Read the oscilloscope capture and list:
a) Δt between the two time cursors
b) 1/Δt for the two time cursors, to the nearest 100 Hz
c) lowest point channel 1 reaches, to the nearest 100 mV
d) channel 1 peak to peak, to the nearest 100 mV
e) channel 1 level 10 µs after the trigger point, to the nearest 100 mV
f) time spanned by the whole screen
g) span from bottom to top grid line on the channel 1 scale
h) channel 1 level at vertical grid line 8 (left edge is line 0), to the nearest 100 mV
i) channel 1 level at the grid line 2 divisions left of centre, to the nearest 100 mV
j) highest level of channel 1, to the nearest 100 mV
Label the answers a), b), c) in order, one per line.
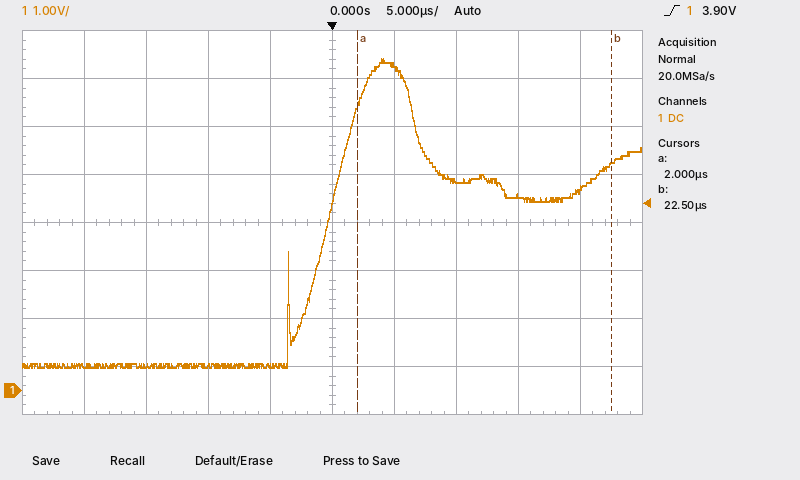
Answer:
a) 20.5 µs
b) 48.8 kHz
c) 500 mV
d) 6.4 V
e) 4.4 V
f) 50 µs
g) 8 V
h) 4.1 V
i) 500 mV
j) 6.9 V
